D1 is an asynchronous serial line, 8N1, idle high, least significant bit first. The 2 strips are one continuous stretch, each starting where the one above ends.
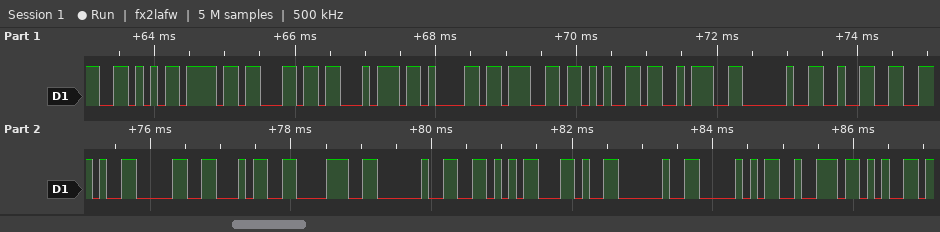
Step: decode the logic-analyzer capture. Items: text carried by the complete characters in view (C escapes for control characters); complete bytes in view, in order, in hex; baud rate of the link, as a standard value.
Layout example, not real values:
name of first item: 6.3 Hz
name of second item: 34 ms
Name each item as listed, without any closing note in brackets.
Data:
text carried by the complete characters in view: "Voltage: 2.048 V, Pre"
complete bytes in view, in order, in hex: 0x56 0x6F 0x6C 0x74 0x61 0x67 0x65 0x3A 0x20 0x32 0x2E 0x30 0x34 0x38 0x20 0x56 0x2C 0x20 0x50 0x72 0x65
baud rate of the link, as a standard value: 9600 baud
